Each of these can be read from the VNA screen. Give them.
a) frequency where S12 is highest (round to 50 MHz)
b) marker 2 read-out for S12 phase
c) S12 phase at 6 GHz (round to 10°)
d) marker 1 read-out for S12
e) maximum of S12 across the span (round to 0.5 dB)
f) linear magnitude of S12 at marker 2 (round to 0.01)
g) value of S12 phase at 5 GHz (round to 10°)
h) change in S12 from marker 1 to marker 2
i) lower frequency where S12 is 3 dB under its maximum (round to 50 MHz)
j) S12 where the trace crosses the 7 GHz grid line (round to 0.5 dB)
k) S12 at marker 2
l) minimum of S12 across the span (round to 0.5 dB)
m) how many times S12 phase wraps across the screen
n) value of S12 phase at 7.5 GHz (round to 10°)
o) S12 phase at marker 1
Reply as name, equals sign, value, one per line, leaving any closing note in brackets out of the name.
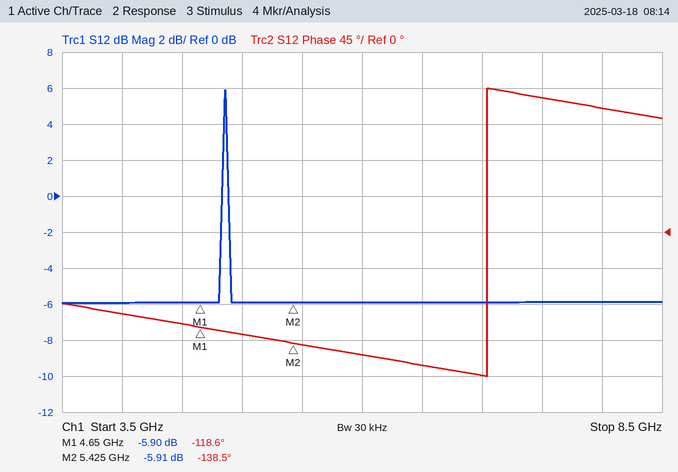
frequency where S12 is highest = 4.85 GHz
marker 2 read-out for S12 phase = -138.5°
S12 phase at 6 GHz = -150°
marker 1 read-out for S12 = -5.90 dB
maximum of S12 across the span = 6.0 dB
linear magnitude of S12 at marker 2 = 0.51
value of S12 phase at 5 GHz = -130°
change in S12 from marker 1 to marker 2 = -0.01 dB
lower frequency where S12 is 3 dB under its maximum = 4.85 GHz
S12 where the trace crosses the 7 GHz grid line = -6.0 dB
S12 at marker 2 = -5.91 dB
minimum of S12 across the span = -6.0 dB
how many times S12 phase wraps across the screen = 1
value of S12 phase at 7.5 GHz = 170°
S12 phase at marker 1 = -118.6°
